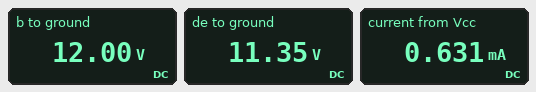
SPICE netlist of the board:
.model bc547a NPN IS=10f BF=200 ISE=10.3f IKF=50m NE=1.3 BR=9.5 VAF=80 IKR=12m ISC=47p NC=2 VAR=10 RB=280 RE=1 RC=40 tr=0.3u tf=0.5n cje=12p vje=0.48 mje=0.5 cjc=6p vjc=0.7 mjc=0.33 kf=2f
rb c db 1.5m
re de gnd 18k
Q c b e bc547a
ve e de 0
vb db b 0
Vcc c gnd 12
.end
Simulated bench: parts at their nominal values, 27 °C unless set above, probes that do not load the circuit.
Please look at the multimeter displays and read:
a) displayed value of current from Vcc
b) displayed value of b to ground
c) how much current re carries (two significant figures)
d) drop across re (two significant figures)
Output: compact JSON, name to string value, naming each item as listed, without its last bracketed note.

{"displayed value of current from Vcc": "0.631 mA", "displayed value of b to ground": "12.00 V", "how much current re carries": "630 µA", "drop across re": "11 V"}
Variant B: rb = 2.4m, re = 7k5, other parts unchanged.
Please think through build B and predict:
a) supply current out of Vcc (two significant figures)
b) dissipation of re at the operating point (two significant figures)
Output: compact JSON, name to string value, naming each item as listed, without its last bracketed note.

{"supply current out of Vcc": "1.5 mA", "dissipation of re at the operating point": "17 mW"}
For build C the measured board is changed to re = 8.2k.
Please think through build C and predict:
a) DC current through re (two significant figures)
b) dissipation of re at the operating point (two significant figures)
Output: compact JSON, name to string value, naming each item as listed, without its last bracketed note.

{"DC current through re": "1.4 mA", "dissipation of re at the operating point": "16 mW"}
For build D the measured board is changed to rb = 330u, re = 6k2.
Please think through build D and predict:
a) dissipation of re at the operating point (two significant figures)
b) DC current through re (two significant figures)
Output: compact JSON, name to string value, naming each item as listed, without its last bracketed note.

{"dissipation of re at the operating point": "21 mW", "DC current through re": "1.8 mA"}
